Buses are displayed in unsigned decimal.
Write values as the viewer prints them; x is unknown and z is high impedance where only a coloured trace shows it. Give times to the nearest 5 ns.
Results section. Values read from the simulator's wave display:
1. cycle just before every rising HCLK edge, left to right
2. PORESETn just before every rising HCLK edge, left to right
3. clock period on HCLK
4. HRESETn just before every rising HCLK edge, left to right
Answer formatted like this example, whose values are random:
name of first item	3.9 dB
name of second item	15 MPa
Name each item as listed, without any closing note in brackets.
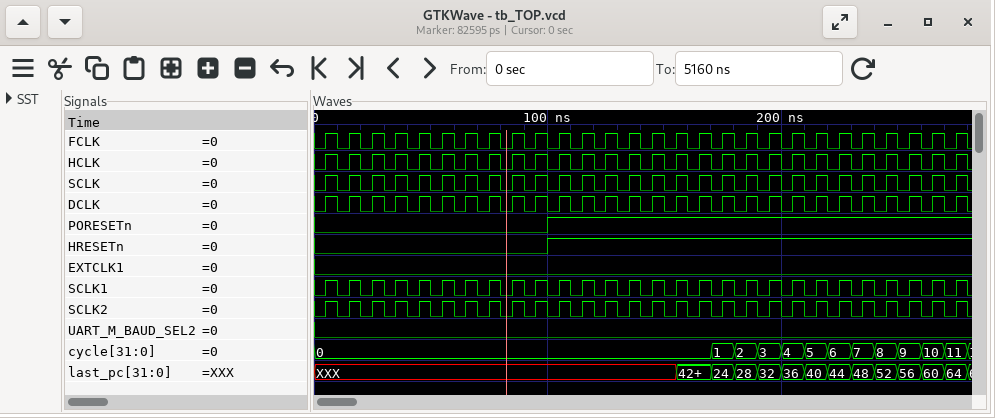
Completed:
cycle just before every rising HCLK edge, left to right	0, 0, 0, 0, 0, 0, 0, 0, 0, 0, 0, 0, 0, 0, 0, 0, 0, 1, 2, 3, 4, 5, 6, 7, 8, 9, 10, 11
PORESETn just before every rising HCLK edge, left to right	0 0 0 0 0 0 0 0 0 0 1 1 1 1 1 1 1 1 1 1 1 1 1 1 1 1 1 1
clock period on HCLK	10 ns
HRESETn just before every rising HCLK edge, left to right	0 0 0 0 0 0 0 0 0 0 1 1 1 1 1 1 1 1 1 1 1 1 1 1 1 1 1 1
